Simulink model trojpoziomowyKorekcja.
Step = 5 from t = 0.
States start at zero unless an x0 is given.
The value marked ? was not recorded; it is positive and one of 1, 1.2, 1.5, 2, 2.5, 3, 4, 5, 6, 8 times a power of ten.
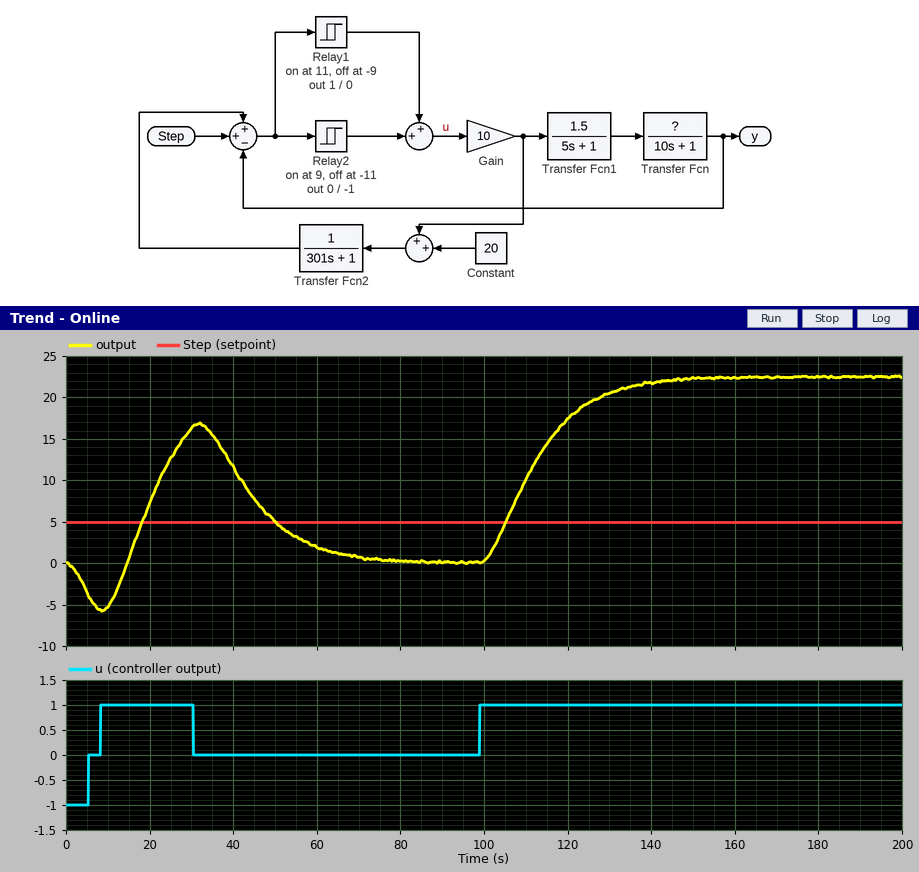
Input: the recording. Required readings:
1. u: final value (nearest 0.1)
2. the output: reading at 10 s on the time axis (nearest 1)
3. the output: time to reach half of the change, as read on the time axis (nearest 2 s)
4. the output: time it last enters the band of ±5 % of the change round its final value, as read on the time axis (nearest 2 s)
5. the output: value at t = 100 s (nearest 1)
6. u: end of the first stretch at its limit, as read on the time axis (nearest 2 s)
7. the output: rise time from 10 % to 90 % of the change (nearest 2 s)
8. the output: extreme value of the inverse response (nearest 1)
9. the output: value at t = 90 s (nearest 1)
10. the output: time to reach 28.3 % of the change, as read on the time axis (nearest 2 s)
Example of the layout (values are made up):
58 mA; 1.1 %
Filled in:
1.0; -5; 24 s; 136 s; 0; 6 s; 112 s; -6; 0; 20 s
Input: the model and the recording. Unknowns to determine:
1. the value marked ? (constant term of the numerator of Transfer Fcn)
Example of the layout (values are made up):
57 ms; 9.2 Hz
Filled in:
1.5
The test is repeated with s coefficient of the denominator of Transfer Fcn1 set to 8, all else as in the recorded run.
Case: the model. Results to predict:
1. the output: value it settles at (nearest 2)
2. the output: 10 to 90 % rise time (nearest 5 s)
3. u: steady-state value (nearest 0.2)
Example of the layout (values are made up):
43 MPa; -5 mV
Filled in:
22; 115 s; 1.0
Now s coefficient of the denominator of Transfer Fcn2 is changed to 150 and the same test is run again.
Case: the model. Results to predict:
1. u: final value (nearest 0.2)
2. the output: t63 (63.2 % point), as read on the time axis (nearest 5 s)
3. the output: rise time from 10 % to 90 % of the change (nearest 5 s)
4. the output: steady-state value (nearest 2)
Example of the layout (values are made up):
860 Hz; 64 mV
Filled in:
1.0; 25 s; 25 s; 22
